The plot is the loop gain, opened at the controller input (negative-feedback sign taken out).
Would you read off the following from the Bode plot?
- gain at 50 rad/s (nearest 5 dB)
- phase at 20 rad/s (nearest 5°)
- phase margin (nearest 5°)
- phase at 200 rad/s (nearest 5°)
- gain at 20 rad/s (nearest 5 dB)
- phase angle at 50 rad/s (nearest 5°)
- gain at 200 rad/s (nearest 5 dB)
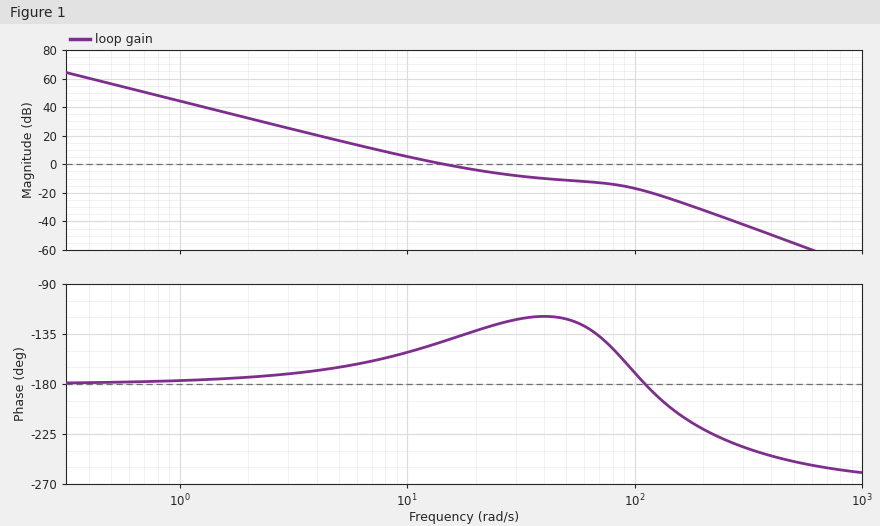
-10 dB
-130°
40°
-220°
-5 dB
-120°
-30 dB
